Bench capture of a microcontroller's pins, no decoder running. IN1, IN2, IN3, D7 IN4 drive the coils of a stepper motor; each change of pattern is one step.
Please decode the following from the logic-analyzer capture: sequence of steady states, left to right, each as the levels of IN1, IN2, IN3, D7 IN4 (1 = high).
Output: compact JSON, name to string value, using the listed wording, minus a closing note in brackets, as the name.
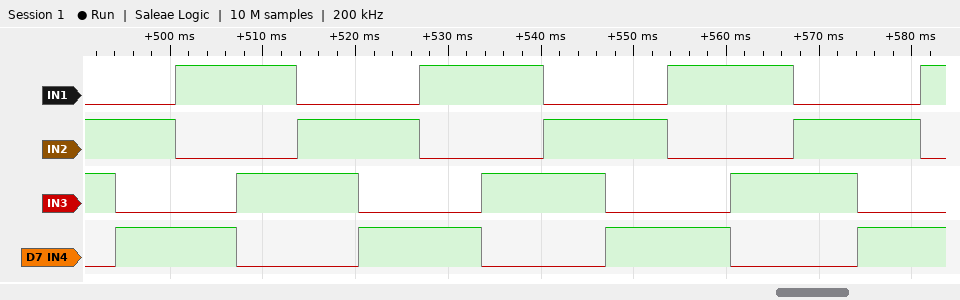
{"sequence of steady states, left to right, each as the levels of IN1, IN2, IN3, D7 IN4": "0110 0101 1001 1010 0110 0101 1001 1010 0110 0101 1001 1010 0110 0101 1001"}
